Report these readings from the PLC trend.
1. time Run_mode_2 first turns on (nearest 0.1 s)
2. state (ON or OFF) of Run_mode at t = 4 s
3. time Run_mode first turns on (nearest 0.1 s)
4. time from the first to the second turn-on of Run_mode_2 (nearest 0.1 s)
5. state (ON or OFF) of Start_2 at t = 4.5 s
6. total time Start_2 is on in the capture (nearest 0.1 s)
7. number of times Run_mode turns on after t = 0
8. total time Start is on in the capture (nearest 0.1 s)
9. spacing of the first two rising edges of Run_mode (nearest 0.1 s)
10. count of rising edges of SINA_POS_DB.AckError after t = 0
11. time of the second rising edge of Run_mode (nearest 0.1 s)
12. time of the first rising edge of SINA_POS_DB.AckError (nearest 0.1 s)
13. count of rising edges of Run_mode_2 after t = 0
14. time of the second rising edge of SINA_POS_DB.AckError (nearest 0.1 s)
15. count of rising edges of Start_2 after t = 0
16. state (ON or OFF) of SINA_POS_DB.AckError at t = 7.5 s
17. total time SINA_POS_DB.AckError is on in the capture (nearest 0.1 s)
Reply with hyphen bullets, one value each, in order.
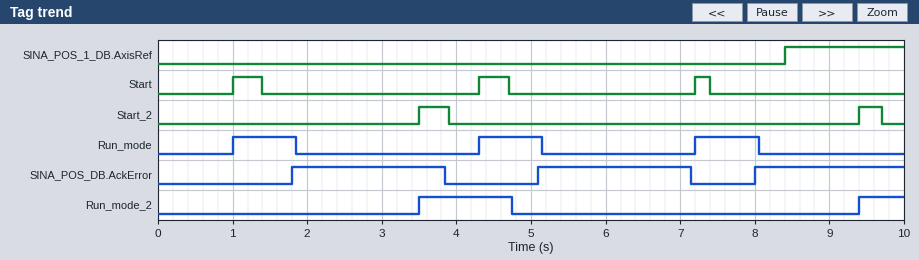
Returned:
- 3.5 s
- OFF
- 1.0 s
- 5.9 s
- OFF
- 0.7 s
- 3
- 1.0 s
- 3.3 s
- 3
- 4.3 s
- 1.8 s
- 2
- 5.1 s
- 2
- OFF
- 6.1 s
